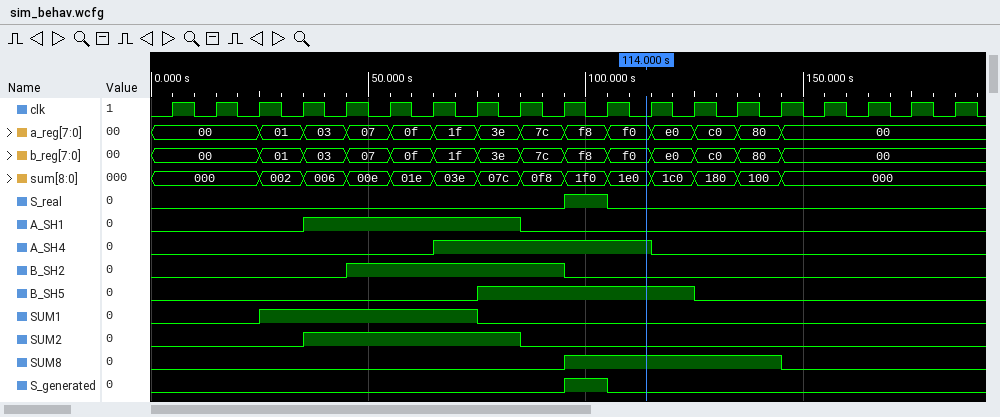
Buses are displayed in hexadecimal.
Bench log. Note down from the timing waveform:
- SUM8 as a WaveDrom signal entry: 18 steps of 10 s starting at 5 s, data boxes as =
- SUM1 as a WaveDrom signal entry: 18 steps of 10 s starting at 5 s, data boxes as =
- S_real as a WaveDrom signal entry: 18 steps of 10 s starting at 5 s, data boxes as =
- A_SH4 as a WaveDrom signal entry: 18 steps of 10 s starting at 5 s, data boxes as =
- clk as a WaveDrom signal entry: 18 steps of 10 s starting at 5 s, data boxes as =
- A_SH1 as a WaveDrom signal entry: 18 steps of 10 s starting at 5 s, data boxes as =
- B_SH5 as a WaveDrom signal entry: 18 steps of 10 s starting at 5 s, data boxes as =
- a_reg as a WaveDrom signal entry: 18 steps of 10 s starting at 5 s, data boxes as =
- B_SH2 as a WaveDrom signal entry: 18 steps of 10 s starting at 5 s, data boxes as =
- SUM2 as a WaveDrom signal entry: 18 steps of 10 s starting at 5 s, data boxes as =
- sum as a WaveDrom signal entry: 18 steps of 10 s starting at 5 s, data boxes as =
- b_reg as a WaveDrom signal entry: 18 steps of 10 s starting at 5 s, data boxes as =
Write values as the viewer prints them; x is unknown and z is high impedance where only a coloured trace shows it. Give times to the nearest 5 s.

{name: 'SUM8', wave: '0........1....0...'}
{name: 'SUM1', wave: '0.1....0..........'}
{name: 'S_real', wave: '0........10.......'}
{name: 'A_SH4', wave: '0.....1....0......'}
{name: 'clk', wave: 'p.................'}
{name: 'A_SH1', wave: '0..1....0.........'}
{name: 'B_SH5', wave: '0......1....0.....'}
{name: 'a_reg', wave: '=.=============...', data: '00 01 03 07 0f 1f 3e 7c f8 f0 e0 c0 80 00'}
{name: 'B_SH2', wave: '0...1....0........'}
{name: 'SUM2', wave: '0..1....0.........'}
{name: 'sum', wave: '=.=============...', data: '000 002 006 00e 01e 03e 07c 0f8 1f0 1e0 1c0 180 100 000'}
{name: 'b_reg', wave: '=.=============...', data: '00 01 03 07 0f 1f 3e 7c f8 f0 e0 c0 80 00'}
